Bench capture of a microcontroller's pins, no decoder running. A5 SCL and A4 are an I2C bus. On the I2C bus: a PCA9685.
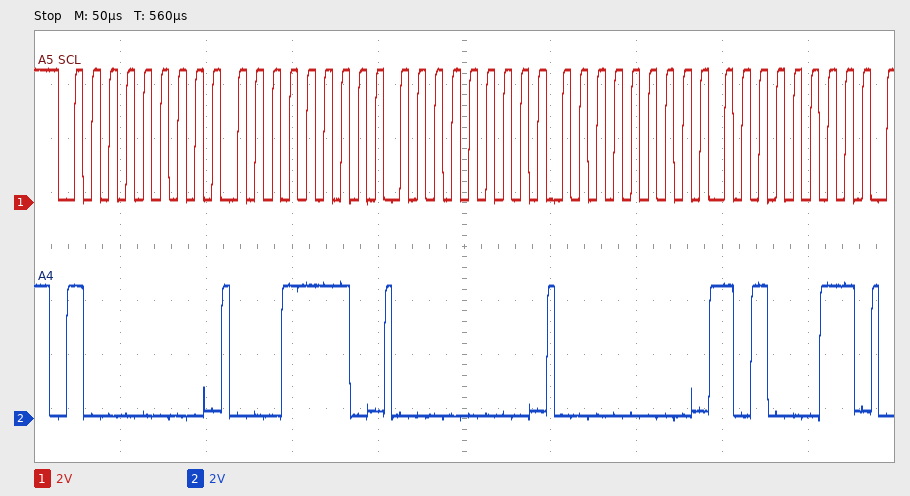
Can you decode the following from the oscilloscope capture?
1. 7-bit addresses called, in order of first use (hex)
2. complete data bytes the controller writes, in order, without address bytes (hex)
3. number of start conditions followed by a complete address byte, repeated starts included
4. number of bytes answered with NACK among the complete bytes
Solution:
0x40
1E 00 00 A3
1
0
